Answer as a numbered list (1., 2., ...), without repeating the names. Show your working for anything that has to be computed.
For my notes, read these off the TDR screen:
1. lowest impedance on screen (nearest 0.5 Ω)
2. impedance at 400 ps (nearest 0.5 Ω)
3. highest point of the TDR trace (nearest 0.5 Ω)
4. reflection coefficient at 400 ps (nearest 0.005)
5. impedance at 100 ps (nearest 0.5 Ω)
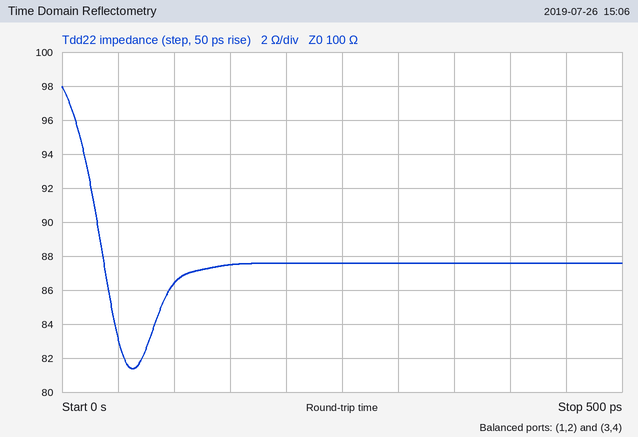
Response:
1. 81.5 Ω
2. 87.5 Ω
3. 98.0 Ω
4. (87.5 − 100)/(87.5 + 100) ≈ -0.0667, so -0.065 to the nearest 0.005
5. 86.5 Ω
